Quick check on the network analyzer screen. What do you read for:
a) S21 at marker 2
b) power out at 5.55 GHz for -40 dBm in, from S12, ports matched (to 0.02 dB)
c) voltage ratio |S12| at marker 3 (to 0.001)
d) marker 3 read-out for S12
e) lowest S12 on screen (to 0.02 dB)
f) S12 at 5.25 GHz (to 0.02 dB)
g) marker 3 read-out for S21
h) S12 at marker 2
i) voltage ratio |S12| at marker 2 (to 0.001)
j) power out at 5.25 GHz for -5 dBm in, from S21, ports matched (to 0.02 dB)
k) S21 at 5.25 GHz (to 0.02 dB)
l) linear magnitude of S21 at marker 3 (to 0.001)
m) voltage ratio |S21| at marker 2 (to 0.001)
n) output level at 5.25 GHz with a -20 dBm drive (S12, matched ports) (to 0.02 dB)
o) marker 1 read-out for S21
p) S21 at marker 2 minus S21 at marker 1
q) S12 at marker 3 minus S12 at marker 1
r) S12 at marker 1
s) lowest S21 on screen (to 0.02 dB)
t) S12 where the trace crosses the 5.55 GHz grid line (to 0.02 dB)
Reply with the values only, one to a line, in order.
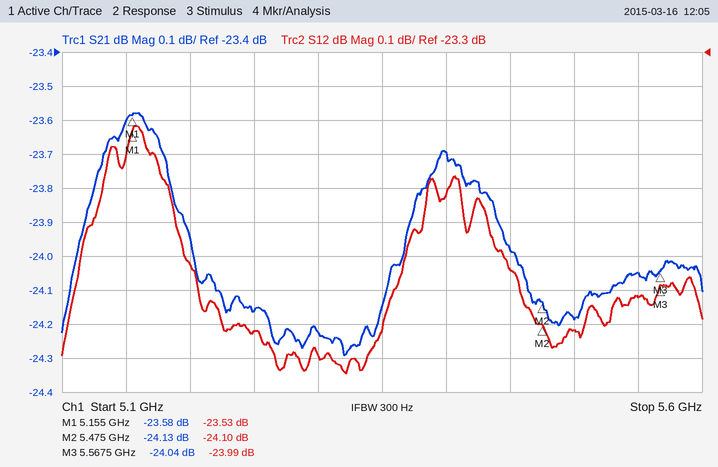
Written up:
-24.13 dB
-64.02 dBm
0.063
-23.99 dB
-24.24 dB
-24.12 dB
-24.04 dB
-24.10 dB
0.062
-29.16 dBm
-24.16 dB
0.063
0.062
-44.12 dBm
-23.58 dB
-0.55 dB
-0.46 dB
-23.53 dB
-24.30 dB
-24.02 dB
